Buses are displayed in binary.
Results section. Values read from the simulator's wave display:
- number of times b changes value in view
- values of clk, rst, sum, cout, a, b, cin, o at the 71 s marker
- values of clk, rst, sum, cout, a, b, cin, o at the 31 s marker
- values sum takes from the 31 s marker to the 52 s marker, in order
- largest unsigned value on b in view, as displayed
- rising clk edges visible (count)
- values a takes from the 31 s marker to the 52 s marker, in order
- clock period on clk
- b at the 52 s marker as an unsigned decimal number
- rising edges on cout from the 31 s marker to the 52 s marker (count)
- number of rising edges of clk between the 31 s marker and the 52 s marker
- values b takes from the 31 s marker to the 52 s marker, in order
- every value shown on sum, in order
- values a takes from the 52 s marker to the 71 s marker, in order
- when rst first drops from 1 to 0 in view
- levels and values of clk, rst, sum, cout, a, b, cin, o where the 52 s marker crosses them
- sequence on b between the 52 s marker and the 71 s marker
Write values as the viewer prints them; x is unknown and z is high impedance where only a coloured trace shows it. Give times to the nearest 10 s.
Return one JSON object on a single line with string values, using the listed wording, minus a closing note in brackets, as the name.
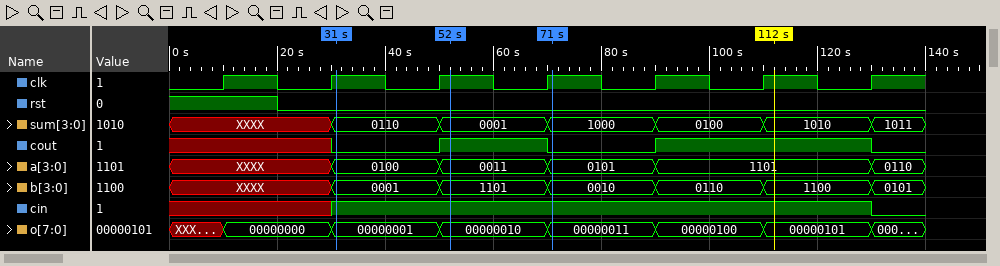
{"number of times b changes value in view": "6", "values of clk, rst, sum, cout, a, b, cin, o at the 71 s marker": "clk=1, rst=0, sum=1000, cout=0, a=0101, b=0010, cin=1, o=00000011", "values of clk, rst, sum, cout, a, b, cin, o at the 31 s marker": "clk=1, rst=0, sum=0110, cout=0, a=0100, b=0001, cin=1, o=00000001", "values sum takes from the 31 s marker to the 52 s marker, in order": "0110, 0001", "largest unsigned value on b in view, as displayed": "1101", "rising clk edges visible": "7", "values a takes from the 31 s marker to the 52 s marker, in order": "0100, 0011", "clock period on clk": "20 s", "b at the 52 s marker as an unsigned decimal number": "13", "rising edges on cout from the 31 s marker to the 52 s marker": "1", "number of rising edges of clk between the 31 s marker and the 52 s marker": "1", "values b takes from the 31 s marker to the 52 s marker, in order": "0001, 1101", "every value shown on sum, in order": "XXXX, 0110, 0001, 1000, 0100, 1010, 1011", "values a takes from the 52 s marker to the 71 s marker, in order": "0011, 0101", "when rst first drops from 1 to 0 in view": "20 s", "levels and values of clk, rst, sum, cout, a, b, cin, o where the 52 s marker crosses them": "clk=1, rst=0, sum=0001, cout=1, a=0011, b=1101, cin=1, o=00000010", "sequence on b between the 52 s marker and the 71 s marker": "1101, 0010"}
